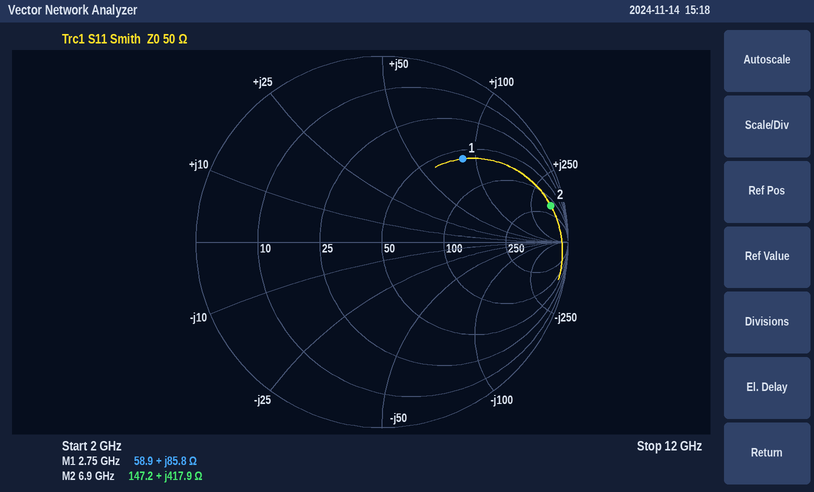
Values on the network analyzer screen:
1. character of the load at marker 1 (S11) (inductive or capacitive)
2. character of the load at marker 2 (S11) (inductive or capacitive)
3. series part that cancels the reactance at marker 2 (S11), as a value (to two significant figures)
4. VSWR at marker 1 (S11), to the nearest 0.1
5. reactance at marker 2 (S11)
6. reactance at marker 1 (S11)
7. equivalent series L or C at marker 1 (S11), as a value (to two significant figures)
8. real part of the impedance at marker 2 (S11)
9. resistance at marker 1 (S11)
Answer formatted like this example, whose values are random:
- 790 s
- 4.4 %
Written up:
- inductive
- inductive
- 55 fF
- 4.3
- +417.9 Ω
- +85.8 Ω
- 5.0 nH
- 147.2 Ω
- 58.9 Ω
